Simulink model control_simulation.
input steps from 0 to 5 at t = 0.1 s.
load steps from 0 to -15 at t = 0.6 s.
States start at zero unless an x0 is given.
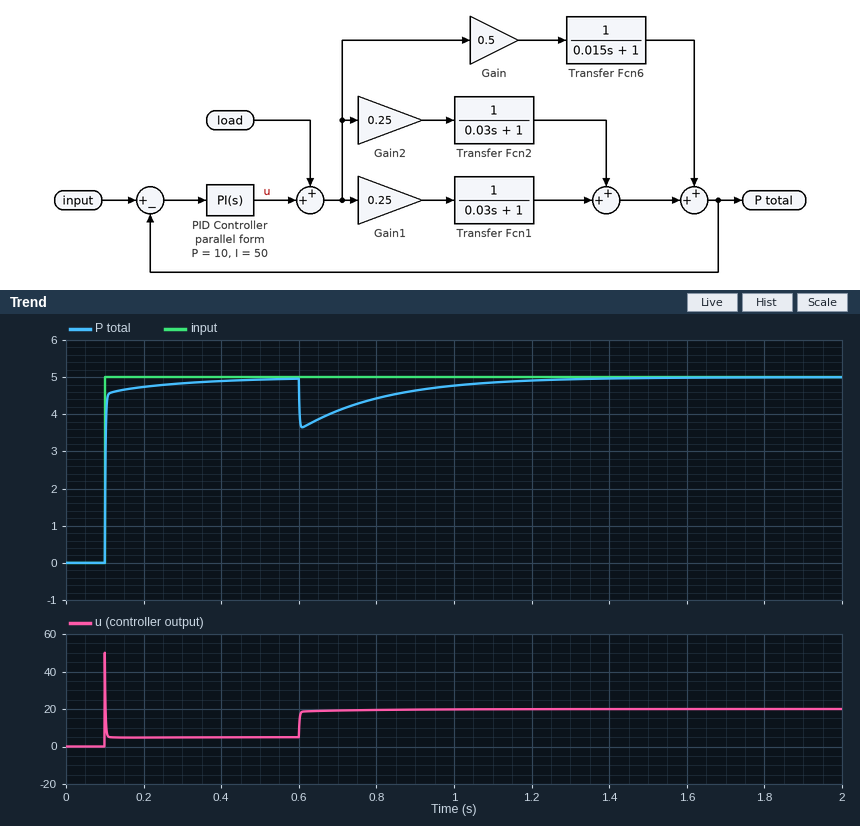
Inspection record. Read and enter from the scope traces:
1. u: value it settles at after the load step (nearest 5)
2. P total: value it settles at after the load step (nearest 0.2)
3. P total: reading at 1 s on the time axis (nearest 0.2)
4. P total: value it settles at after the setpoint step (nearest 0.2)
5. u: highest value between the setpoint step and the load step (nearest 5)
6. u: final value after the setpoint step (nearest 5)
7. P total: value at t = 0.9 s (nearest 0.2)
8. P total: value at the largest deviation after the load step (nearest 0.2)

20
5.0
4.8
5.0
50
5
4.6
3.6
